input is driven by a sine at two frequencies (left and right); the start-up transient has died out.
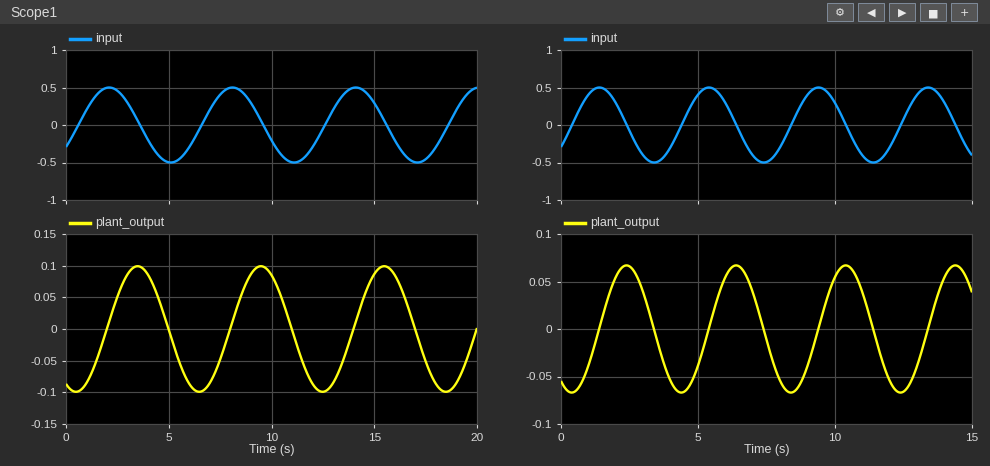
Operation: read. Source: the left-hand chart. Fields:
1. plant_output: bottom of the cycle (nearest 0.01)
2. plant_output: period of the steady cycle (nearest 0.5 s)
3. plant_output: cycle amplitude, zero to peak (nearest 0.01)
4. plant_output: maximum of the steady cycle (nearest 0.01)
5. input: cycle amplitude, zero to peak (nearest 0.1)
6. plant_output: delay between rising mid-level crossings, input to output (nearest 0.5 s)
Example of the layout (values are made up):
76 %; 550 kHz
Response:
-0.10; 6.0 s; 0.10; 0.10; 0.5; 1.5 s
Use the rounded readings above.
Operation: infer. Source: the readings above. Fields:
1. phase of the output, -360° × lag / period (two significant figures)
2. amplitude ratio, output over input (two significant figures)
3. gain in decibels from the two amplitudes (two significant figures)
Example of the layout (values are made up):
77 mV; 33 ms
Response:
-90°; 0.20; -14 dB
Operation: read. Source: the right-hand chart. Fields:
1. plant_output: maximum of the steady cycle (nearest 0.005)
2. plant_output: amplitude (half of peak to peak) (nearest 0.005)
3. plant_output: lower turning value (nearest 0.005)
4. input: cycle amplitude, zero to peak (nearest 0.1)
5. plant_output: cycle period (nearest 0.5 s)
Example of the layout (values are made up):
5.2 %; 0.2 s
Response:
0.065; 0.065; -0.065; 0.5; 4.0 s
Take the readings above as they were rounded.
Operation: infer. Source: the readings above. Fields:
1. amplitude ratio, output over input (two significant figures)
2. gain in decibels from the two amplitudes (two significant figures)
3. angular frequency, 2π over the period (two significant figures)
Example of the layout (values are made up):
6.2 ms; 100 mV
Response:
0.13; -18 dB; 1.6 rad/s
